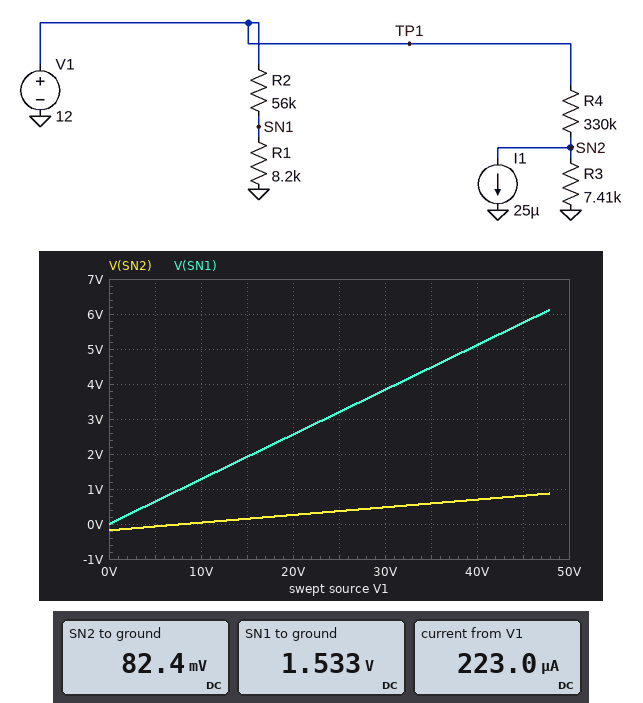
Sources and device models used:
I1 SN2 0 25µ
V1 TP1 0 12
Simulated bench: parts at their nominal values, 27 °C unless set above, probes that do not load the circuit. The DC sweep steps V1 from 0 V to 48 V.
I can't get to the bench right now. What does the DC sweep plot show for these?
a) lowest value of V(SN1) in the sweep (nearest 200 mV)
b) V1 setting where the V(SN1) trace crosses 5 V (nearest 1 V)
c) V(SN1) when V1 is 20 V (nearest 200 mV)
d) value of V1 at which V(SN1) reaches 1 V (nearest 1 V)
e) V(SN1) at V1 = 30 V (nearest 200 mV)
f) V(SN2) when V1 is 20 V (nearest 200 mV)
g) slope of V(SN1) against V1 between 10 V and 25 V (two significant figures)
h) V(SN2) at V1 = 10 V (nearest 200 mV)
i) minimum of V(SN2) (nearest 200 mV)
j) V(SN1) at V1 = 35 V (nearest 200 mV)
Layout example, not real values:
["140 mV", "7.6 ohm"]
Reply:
["0 V", "39 V", "2.6 V", "8 V", "3.8 V", "200 mV", "0.13 V/V", "0 V", "-200 mV", "4.4 V"]
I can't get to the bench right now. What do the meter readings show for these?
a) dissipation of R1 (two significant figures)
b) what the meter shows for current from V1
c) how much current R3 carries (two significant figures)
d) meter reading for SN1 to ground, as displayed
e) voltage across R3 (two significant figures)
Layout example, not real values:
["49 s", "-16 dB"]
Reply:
["290 µW", "223.0 µA", "11 µA", "1.533 V", "82 mV"]
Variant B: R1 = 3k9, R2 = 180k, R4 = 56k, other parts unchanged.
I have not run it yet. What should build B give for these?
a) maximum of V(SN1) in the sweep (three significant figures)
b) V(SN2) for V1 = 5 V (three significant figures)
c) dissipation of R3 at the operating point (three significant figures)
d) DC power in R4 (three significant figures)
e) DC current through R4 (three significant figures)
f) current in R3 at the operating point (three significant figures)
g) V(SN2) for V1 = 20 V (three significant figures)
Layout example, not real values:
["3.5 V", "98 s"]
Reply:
["1.02 V", "421 mV", "207 µW", "2.07 mW", "192 µA", "167 µA", "2.17 V"]
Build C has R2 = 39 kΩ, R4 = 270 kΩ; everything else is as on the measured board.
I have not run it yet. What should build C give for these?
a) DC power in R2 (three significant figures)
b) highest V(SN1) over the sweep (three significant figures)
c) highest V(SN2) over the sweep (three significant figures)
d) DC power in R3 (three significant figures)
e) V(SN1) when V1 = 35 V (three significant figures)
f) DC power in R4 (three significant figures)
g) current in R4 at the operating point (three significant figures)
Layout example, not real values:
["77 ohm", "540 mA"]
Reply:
["2.52 mW", "8.34 V", "1.10 V", "2.65 µW", "6.08 V", "521 µW", "43.9 µA"]
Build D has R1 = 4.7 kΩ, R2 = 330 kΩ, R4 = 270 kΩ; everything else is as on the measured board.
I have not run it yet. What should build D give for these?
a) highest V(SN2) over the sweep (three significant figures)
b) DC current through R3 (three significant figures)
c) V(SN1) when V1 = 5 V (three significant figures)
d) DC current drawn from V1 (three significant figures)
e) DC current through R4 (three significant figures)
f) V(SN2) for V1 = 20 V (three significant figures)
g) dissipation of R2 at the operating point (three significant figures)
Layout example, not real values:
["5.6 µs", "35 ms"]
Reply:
["1.10 V", "18.9 µA", "70.2 mV", "79.8 µA", "43.9 µA", "354 mV", "424 µW"]
